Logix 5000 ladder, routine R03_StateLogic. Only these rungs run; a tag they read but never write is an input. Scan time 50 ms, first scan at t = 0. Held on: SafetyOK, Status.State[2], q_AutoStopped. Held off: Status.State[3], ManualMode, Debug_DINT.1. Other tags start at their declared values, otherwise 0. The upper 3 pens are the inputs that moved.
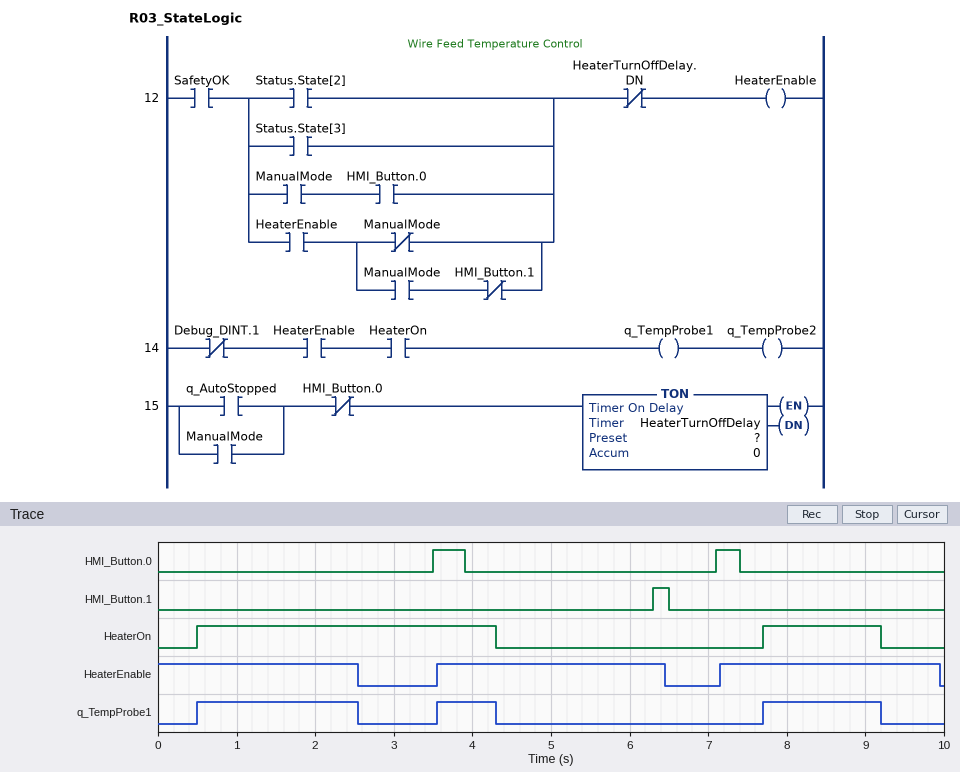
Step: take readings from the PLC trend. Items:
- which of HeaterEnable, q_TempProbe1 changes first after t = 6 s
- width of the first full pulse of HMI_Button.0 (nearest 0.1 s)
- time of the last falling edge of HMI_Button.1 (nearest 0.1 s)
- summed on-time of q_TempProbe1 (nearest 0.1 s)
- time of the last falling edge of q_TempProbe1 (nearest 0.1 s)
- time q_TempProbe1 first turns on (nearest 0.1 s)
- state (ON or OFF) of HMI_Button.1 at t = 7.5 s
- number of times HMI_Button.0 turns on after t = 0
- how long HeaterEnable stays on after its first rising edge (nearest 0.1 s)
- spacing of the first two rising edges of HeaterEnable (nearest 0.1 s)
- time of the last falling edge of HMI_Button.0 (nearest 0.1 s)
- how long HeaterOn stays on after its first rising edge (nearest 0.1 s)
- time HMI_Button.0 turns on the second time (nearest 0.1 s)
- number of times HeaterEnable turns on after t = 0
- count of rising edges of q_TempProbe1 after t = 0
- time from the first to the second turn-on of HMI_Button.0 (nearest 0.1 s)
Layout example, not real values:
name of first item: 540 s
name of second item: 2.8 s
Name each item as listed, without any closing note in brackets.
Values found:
which of HeaterEnable, q_TempProbe1 changes first after t = 6 s: HeaterEnable
width of the first full pulse of HMI_Button.0: 0.4 s
time of the last falling edge of HMI_Button.1: 6.5 s
summed on-time of q_TempProbe1: 4.3 s
time of the last falling edge of q_TempProbe1: 9.2 s
time q_TempProbe1 first turns on: 0.5 s
state (ON or OFF) of HMI_Button.1 at t = 7.5 s: OFF
number of times HMI_Button.0 turns on after t = 0: 2
how long HeaterEnable stays on after its first rising edge: 2.9 s
spacing of the first two rising edges of HeaterEnable: 3.6 s
time of the last falling edge of HMI_Button.0: 7.4 s
how long HeaterOn stays on after its first rising edge: 3.8 s
time HMI_Button.0 turns on the second time: 7.1 s
number of times HeaterEnable turns on after t = 0: 2
count of rising edges of q_TempProbe1 after t = 0: 3
time from the first to the second turn-on of HMI_Button.0: 3.6 s
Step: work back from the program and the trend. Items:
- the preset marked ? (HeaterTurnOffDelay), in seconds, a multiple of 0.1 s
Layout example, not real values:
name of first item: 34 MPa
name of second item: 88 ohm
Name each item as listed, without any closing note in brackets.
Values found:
the preset marked ? (HeaterTurnOffDelay), in seconds, a multiple of 0.1 s: 2.5 s
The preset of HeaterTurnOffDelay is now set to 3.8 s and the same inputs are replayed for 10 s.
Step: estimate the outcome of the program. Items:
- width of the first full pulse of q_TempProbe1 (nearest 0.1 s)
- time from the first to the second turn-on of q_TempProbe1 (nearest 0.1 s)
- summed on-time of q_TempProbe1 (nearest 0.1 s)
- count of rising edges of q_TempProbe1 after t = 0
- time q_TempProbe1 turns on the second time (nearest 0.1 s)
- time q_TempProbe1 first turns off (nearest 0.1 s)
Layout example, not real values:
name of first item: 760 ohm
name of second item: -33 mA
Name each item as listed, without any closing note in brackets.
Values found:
width of the first full pulse of q_TempProbe1: 3.8 s
time from the first to the second turn-on of q_TempProbe1: 7.2 s
summed on-time of q_TempProbe1: 5.3 s
count of rising edges of q_TempProbe1 after t = 0: 2
time q_TempProbe1 turns on the second time: 7.7 s
time q_TempProbe1 first turns off: 4.3 s
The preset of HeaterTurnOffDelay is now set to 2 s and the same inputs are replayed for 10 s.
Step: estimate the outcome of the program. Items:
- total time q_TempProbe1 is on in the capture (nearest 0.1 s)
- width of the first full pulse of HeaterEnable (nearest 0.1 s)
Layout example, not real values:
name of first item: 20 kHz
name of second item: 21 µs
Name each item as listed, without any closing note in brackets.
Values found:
total time q_TempProbe1 is on in the capture: 3.8 s
width of the first full pulse of HeaterEnable: 2.4 s
